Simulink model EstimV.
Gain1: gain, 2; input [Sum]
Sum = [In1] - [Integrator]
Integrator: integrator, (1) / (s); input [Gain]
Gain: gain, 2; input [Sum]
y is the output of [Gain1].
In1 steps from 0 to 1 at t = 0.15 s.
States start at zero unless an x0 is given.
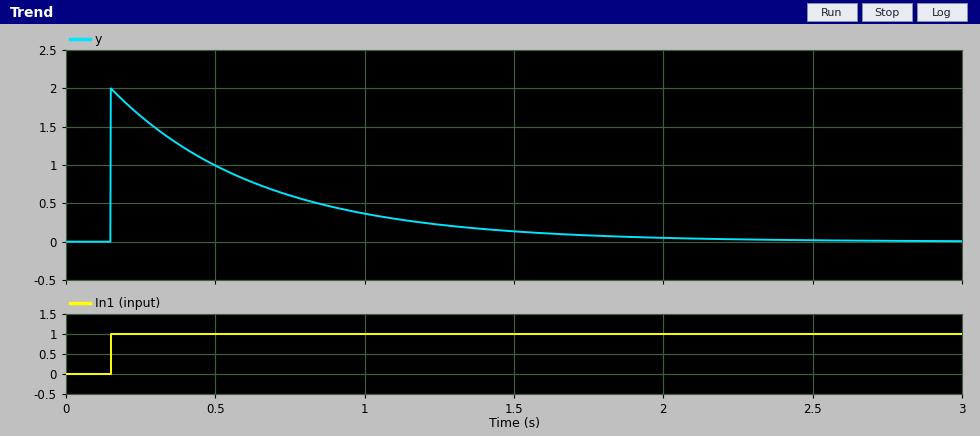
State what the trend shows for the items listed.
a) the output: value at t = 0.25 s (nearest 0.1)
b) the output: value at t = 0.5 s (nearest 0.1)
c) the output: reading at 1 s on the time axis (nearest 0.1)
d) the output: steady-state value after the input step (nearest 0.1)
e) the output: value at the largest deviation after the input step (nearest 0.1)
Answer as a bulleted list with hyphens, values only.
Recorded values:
- 1.6
- 1.0
- 0.4
- 0.0
- 2.0
